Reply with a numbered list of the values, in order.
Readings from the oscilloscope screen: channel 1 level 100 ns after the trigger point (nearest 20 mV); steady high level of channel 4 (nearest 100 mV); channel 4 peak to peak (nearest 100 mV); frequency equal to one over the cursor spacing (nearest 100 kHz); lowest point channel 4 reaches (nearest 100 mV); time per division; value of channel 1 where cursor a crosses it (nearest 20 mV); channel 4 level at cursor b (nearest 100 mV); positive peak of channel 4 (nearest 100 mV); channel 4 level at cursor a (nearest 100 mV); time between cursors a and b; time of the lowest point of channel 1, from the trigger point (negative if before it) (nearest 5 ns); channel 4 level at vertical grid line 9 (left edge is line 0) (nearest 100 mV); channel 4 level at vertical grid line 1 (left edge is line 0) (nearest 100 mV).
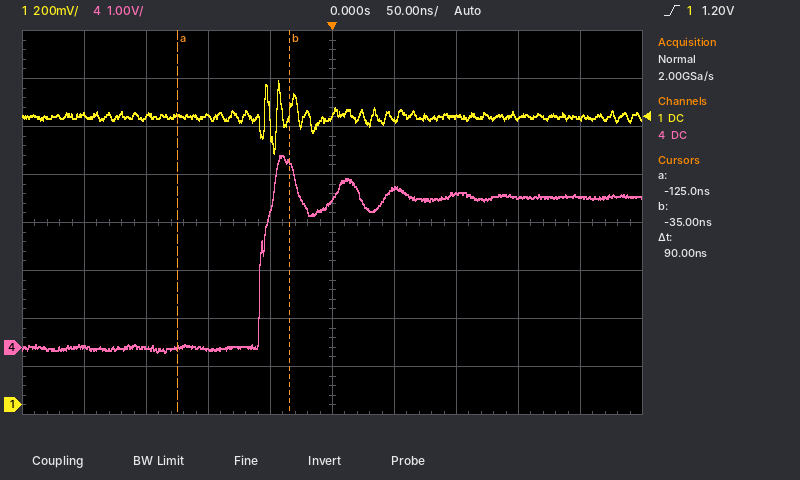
1. 1.20 V
2. 3.1 V
3. 4.1 V
4. 11.1 MHz
5. -100 mV
6. 50 ns
7. 1.20 V
8. 3.8 V
9. 4.0 V
10. 0.0 V
11. 90 ns
12. -45 ns
13. 3.1 V
14. 0.0 V
